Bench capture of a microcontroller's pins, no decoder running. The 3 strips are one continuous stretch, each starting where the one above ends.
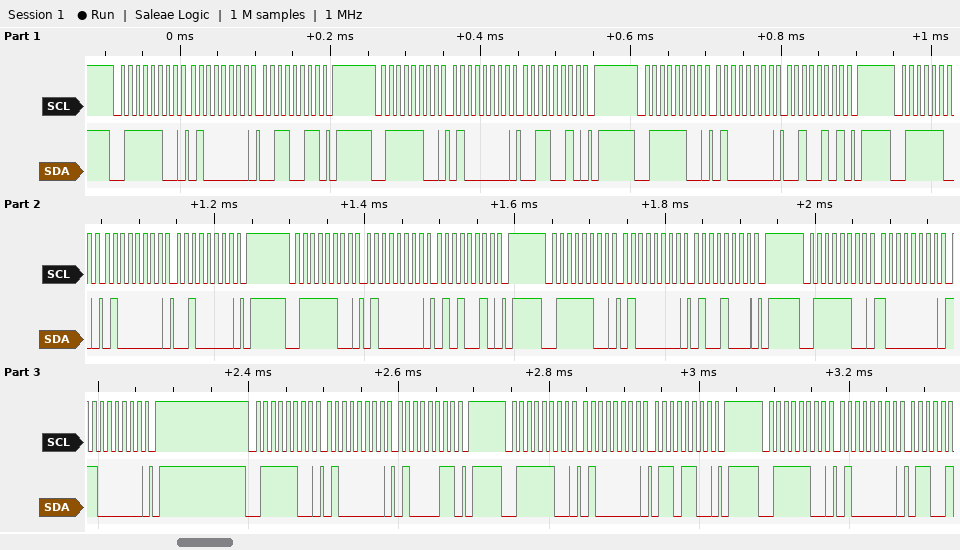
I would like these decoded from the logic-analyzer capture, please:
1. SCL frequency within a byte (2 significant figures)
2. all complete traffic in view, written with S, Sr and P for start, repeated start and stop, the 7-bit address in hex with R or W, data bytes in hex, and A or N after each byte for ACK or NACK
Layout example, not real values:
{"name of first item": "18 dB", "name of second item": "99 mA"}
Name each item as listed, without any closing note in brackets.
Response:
{"SCL frequency within a byte": "100 kHz", "all complete traffic in view, written with S, Sr and P for start, repeated start and stop, the 7-bit address in hex with R or W, data bytes in hex, and A or N after each byte for ACK or NACK": "S 3EW A 40 A 33 A P S 3EW A 40 A 32 A P S 3EW A 40 A 25 A P S 3EW A 40 A 20 A P S 3EW A 40 A 52 A P S 3EW A 40 A 48 A P S 3EW A 80 A C0 A P S 3EW A 40 A 43 A P S 3EW A 40 A 6C A P S 3EW A 40 A"}
